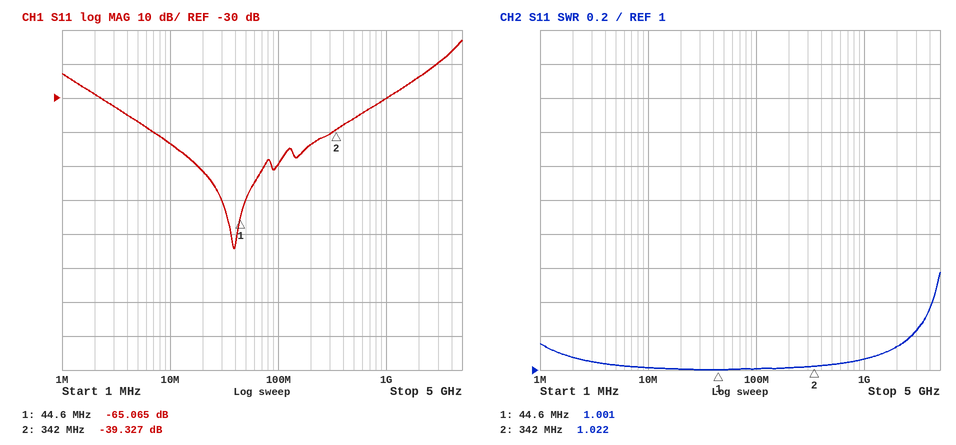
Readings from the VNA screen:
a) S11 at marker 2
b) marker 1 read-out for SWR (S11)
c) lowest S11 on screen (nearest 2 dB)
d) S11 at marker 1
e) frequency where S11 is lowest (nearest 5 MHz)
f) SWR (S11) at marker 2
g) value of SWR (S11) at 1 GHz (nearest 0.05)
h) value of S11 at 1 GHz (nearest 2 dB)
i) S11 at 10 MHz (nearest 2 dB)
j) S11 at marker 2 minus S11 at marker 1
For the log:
-39.327 dB
1.001
-74 dB
-65.065 dB
40 MHz
1.022
1.05
-30 dB
-44 dB
25.738 dB
